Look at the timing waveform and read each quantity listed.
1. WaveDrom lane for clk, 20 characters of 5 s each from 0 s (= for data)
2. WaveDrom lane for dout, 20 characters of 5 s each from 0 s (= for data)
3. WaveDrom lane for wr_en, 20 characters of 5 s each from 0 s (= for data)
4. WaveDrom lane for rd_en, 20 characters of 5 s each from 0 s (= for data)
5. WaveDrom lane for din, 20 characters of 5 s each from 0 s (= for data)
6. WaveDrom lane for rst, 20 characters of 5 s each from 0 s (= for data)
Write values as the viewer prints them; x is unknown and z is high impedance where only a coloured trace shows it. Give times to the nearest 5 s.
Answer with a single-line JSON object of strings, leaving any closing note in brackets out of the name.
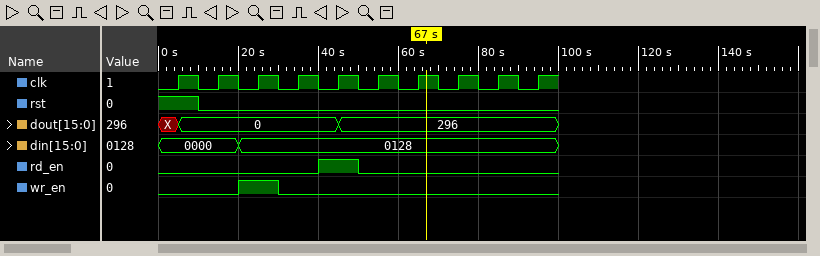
{"WaveDrom lane for clk, 20 characters of 5 s each from 0 s": "{name: 'clk', wave: '01010101010101010101'}", "WaveDrom lane for dout, 20 characters of 5 s each from 0 s": "{name: 'dout', wave: 'x=.......=..........', data: '0 296'}", "WaveDrom lane for wr_en, 20 characters of 5 s each from 0 s": "{name: 'wr_en', wave: '0...1.0.............'}", "WaveDrom lane for rd_en, 20 characters of 5 s each from 0 s": "{name: 'rd_en', wave: '0.......1.0.........'}", "WaveDrom lane for din, 20 characters of 5 s each from 0 s": "{name: 'din', wave: '=...=...............', data: '0000 0128'}", "WaveDrom lane for rst, 20 characters of 5 s each from 0 s": "{name: 'rst', wave: '1.0.................'}"}
